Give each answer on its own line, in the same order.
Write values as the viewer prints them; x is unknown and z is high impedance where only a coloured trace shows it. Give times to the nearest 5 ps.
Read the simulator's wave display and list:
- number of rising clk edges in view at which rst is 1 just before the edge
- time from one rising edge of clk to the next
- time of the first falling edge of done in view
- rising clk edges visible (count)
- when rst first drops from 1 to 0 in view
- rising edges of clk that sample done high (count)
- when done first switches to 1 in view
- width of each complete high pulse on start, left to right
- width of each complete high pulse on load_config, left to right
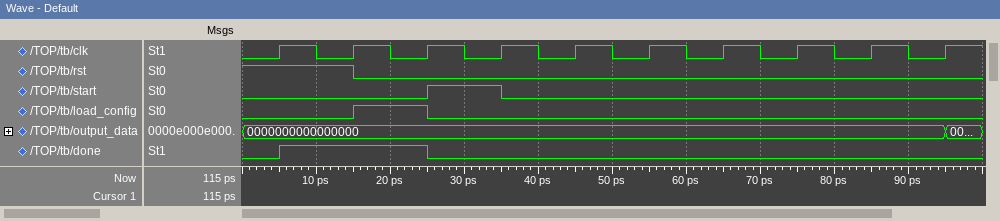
2
10 ps
25 ps
10
15 ps
2
5 ps
10 ps
10 ps
